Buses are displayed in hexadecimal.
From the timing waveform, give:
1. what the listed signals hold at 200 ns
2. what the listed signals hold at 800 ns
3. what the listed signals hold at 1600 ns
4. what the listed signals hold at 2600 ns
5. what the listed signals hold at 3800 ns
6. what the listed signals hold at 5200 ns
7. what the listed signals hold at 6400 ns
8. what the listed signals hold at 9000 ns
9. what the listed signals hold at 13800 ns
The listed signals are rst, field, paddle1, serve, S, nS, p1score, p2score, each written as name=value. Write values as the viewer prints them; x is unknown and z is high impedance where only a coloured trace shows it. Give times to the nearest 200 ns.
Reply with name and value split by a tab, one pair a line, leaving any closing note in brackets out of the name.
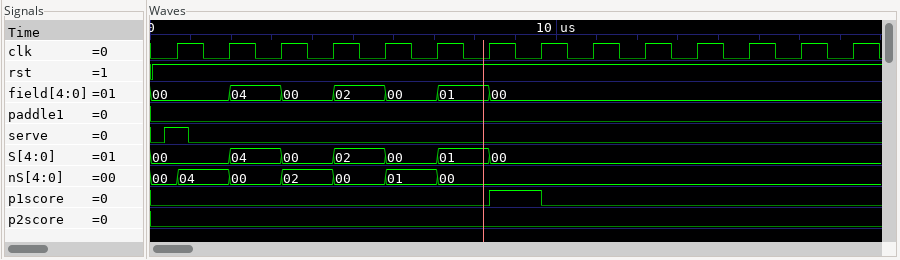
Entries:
what the listed signals hold at 200 ns	rst=1, field=00, paddle1=0, serve=0, S=00, nS=00, p1score=0, p2score=0
what the listed signals hold at 800 ns	rst=1, field=00, paddle1=0, serve=1, S=00, nS=04, p1score=0, p2score=0
what the listed signals hold at 1600 ns	rst=1, field=00, paddle1=0, serve=0, S=00, nS=04, p1score=0, p2score=0
what the listed signals hold at 2600 ns	rst=1, field=04, paddle1=0, serve=0, S=04, nS=00, p1score=0, p2score=0
what the listed signals hold at 3800 ns	rst=1, field=00, paddle1=0, serve=0, S=00, nS=02, p1score=0, p2score=0
what the listed signals hold at 5200 ns	rst=1, field=02, paddle1=0, serve=0, S=02, nS=00, p1score=0, p2score=0
what the listed signals hold at 6400 ns	rst=1, field=00, paddle1=0, serve=0, S=00, nS=01, p1score=0, p2score=0
what the listed signals hold at 9000 ns	rst=1, field=00, paddle1=0, serve=0, S=00, nS=00, p1score=1, p2score=0
what the listed signals hold at 13800 ns	rst=1, field=00, paddle1=0, serve=0, S=00, nS=00, p1score=0, p2score=0
